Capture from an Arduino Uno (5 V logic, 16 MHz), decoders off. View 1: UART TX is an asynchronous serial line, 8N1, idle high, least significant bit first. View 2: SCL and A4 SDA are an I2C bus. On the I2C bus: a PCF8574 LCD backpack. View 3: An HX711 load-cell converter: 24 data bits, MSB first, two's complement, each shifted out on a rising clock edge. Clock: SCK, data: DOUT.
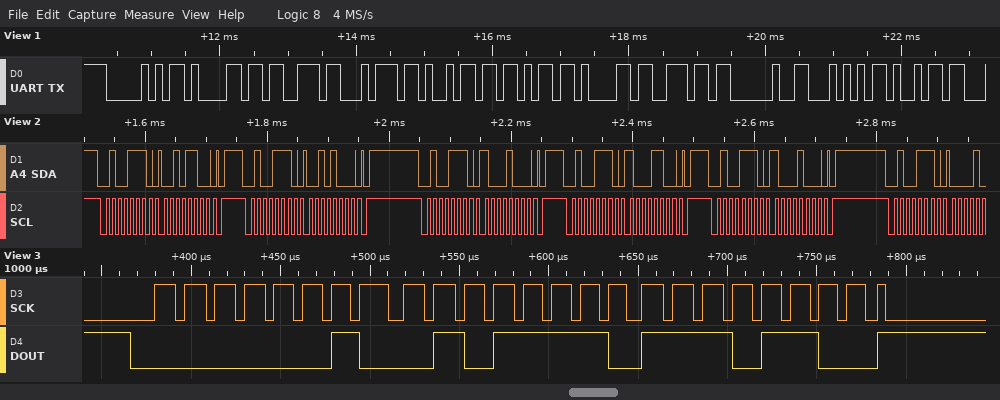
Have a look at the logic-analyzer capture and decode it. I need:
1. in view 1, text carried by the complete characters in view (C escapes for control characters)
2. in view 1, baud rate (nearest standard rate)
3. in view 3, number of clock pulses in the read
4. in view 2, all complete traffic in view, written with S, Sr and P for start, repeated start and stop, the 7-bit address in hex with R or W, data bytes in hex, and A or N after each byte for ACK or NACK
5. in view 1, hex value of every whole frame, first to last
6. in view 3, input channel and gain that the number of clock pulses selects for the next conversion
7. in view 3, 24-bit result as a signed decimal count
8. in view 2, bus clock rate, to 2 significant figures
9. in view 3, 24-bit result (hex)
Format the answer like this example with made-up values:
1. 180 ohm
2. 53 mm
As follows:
1. "Pastikan Ti"
2. 9600 baud
3. 25
4. S 27W A 2C A P S 27W A 28 A P S 27W A 88 A P S 27W A 8C A P S 27W A 88 A P S 27W A
5. 0x50 0x61 0x73 0x74 0x69 0x6B 0x61 0x6E 0x20 0x54 0x69
6. channel A, gain 128
7. 155372
8. 100 kHz
9. 0x025EEC
